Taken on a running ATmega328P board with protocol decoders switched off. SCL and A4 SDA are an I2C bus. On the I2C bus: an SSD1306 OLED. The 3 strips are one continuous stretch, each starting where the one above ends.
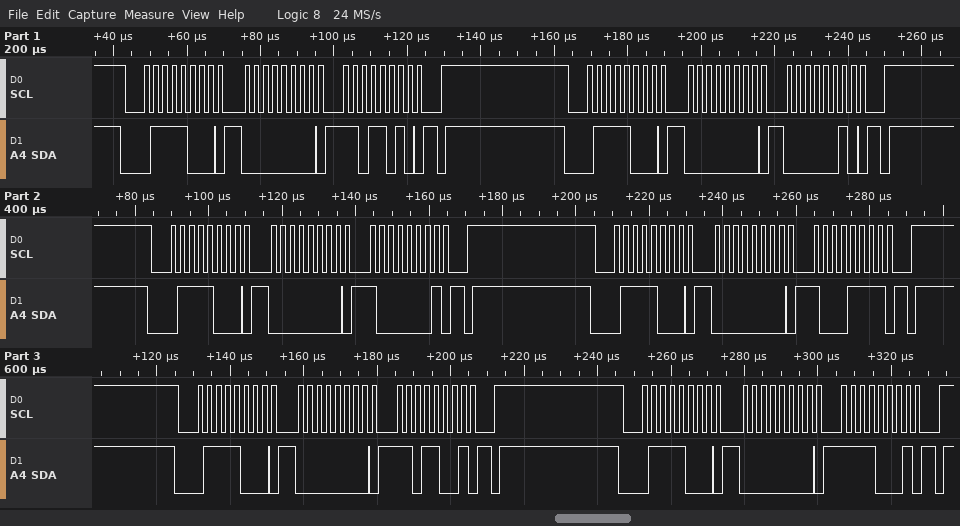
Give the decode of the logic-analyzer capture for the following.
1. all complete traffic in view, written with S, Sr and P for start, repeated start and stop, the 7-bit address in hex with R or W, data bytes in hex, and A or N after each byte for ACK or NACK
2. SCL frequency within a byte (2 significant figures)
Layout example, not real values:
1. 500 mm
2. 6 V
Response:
1. S 3CW A 00 A DA A P S 3CW A 00 A 02 A P S 3CW A 00 A 81 A P S 3CW A 00 A 8F A P S 3CW A 00 A D9 A P S 3CW A 00 A F1 A P
2. 400 kHz
